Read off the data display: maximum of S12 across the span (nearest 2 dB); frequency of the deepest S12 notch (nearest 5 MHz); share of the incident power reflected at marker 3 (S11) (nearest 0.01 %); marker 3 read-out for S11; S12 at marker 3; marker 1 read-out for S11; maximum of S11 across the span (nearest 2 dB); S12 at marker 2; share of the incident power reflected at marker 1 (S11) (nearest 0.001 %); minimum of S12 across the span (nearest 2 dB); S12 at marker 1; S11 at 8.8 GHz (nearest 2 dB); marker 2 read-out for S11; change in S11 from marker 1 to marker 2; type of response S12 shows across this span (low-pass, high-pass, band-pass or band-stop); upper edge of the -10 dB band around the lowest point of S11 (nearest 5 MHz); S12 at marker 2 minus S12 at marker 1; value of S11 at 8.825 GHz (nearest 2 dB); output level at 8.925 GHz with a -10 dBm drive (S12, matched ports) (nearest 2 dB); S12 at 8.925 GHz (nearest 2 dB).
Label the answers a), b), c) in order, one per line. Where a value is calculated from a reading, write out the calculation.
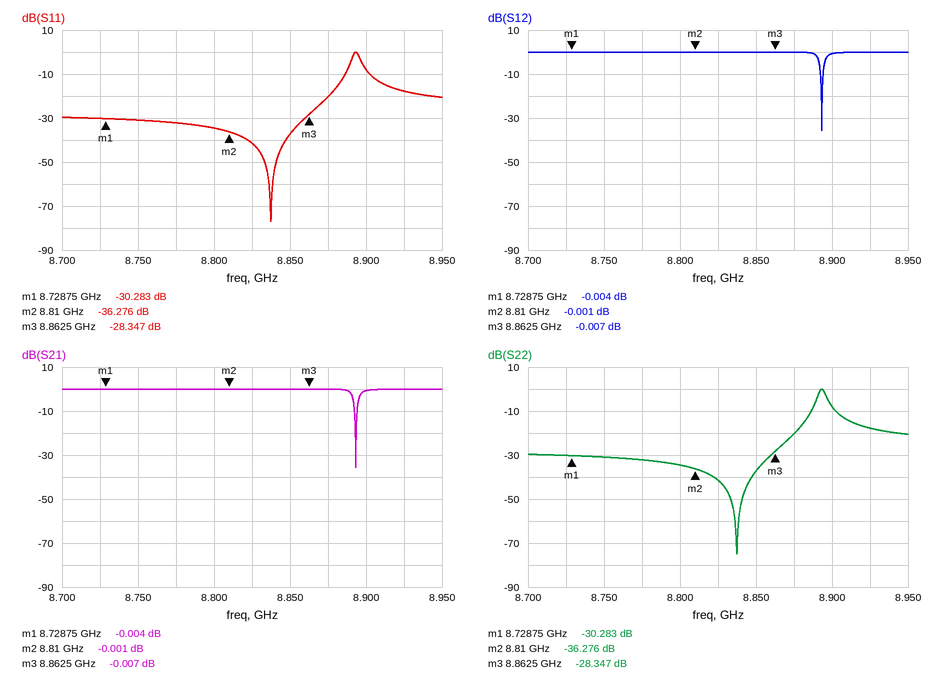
a) 0 dB
b) 8.895 GHz
c) 10^(-28.347/10) ≈ 0.15 %
d) -28.347 dB
e) -0.007 dB
f) -30.283 dB
g) 0 dB
h) -0.001 dB
i) 10^(-30.283/10) ≈ 0.094 %
j) -36 dB
k) -0.004 dB
l) -34 dB
m) -36.276 dB
n) -36.276 − (-30.283) = -5.993 dB
o) band-stop
p) 8.885 GHz
q) -0.001 − (-0.004) = 0.003 dB
r) -42 dB
s) -10 dBm + (0 dB) = -10 dBm
t) 0 dB
